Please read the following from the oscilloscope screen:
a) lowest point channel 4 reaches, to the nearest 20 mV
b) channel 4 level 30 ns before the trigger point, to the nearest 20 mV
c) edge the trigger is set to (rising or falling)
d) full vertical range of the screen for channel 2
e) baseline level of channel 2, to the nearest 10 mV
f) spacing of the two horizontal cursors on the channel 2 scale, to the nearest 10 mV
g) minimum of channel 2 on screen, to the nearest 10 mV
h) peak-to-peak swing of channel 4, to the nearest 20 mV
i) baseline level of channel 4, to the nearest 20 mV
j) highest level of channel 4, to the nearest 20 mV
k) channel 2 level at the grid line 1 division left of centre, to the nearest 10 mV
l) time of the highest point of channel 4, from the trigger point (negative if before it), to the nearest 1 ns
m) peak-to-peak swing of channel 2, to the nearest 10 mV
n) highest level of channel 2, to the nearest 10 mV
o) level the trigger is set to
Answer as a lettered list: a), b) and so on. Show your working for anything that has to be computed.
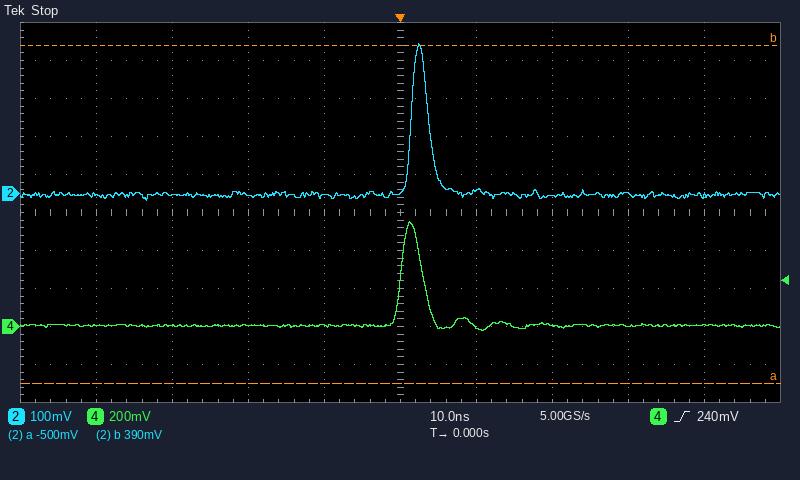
a) -20 mV
b) 0 mV
c) rising
d) 1 V
e) 0 mV
f) 890 mV
g) -20 mV
h) 560 mV − (-20 mV) = 580 mV
i) 0 mV
j) 560 mV
k) -10 mV
l) +1 ns
m) 390 mV − (-20 mV) = 410 mV
n) 390 mV
o) 240 mV
